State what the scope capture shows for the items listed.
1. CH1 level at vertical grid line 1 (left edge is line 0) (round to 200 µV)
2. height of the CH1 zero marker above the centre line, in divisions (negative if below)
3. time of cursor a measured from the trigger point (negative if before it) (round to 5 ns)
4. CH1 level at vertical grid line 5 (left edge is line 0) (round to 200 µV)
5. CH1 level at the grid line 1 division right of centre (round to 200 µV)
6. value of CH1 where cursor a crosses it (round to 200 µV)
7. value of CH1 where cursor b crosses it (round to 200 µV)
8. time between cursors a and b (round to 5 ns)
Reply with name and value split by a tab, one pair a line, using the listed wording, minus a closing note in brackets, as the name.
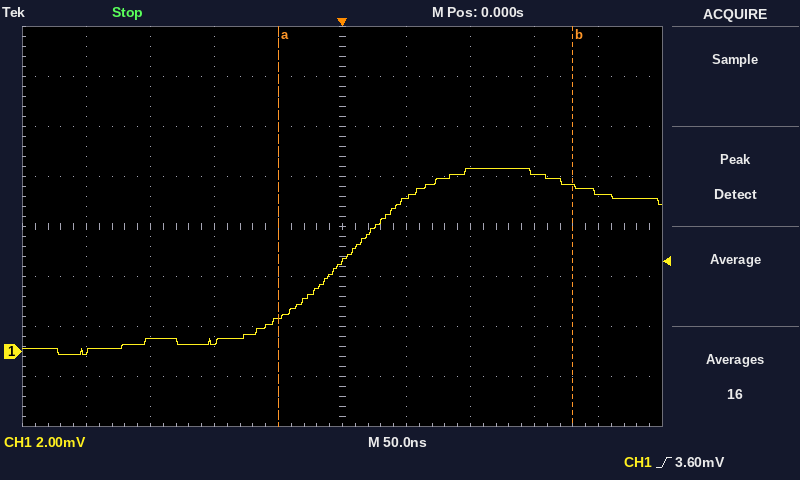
CH1 level at vertical grid line 1 (left edge is line 0)	0.0 mV
height of the CH1 zero marker above the centre line, in divisions	-2.5 div
time of cursor a measured from the trigger point (negative if before it)	-50 ns
CH1 level at vertical grid line 5 (left edge is line 0)	3.6 mV
CH1 level at the grid line 1 division right of centre	6.2 mV
value of CH1 where cursor a crosses it	1.4 mV
value of CH1 where cursor b crosses it	6.6 mV
time between cursors a and b	230 ns
